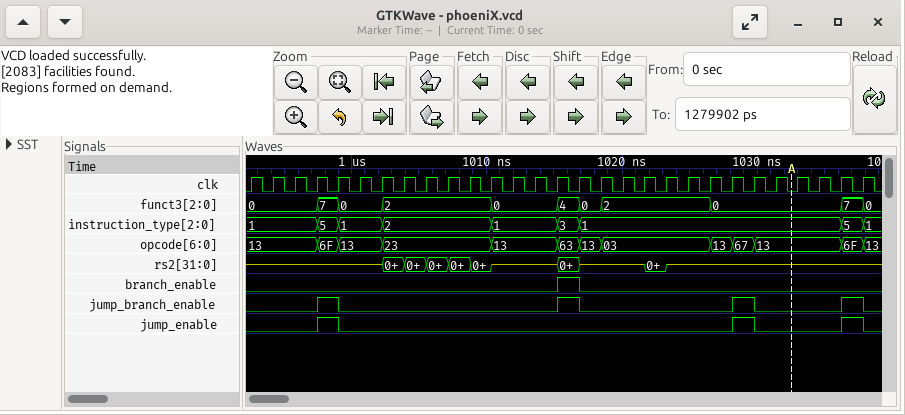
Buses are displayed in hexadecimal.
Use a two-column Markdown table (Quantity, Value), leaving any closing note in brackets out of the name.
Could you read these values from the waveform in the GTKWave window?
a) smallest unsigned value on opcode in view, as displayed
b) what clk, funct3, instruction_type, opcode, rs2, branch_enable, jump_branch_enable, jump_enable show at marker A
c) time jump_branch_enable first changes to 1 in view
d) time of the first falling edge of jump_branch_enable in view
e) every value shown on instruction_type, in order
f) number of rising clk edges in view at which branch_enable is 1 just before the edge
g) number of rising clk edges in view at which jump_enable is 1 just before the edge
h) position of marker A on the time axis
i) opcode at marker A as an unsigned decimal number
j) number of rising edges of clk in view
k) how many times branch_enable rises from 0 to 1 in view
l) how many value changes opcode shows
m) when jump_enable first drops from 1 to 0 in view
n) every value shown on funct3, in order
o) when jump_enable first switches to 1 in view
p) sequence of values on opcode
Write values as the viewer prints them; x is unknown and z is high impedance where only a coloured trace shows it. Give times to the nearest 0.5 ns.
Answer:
| Quantity | Value |
|---|---|
| smallest unsigned value on opcode in view, as displayed | 03 |
| what clk, funct3, instruction_type, opcode, rs2, branch_enable, jump_branch_enable, jump_enable show at marker A | clk=0, funct3=0, instruction_type=1, opcode=13, rs2=z, branch_enable=0, jump_branch_enable=0, jump_enable=0 |
| time jump_branch_enable first changes to 1 in view | 997.5 ns |
| time of the first falling edge of jump_branch_enable in view | 999 ns |
| every value shown on instruction_type, in order | 1, 5, 1, 2, 1, 3, 1, 5, 1 |
| number of rising clk edges in view at which branch_enable is 1 just before the edge | 1 |
| number of rising clk edges in view at which jump_enable is 1 just before the edge | 3 |
| position of marker A on the time axis | 1032.5 ns |
| opcode at marker A as an unsigned decimal number | 19 |
| number of rising edges of clk in view | 29 |
| how many times branch_enable rises from 0 to 1 in view | 1 |
| how many value changes opcode shows | 12 |
| when jump_enable first drops from 1 to 0 in view | 999 ns |
| every value shown on funct3, in order | 0, 7, 0, 2, 0, 4, 0, 2, 0, 7, 0 |
| when jump_enable first switches to 1 in view | 997.5 ns |
| sequence of values on opcode | 13, 6F, 13, 23, 13, 63, 13, 03, 13, 67, 13, 6F, 13 |
